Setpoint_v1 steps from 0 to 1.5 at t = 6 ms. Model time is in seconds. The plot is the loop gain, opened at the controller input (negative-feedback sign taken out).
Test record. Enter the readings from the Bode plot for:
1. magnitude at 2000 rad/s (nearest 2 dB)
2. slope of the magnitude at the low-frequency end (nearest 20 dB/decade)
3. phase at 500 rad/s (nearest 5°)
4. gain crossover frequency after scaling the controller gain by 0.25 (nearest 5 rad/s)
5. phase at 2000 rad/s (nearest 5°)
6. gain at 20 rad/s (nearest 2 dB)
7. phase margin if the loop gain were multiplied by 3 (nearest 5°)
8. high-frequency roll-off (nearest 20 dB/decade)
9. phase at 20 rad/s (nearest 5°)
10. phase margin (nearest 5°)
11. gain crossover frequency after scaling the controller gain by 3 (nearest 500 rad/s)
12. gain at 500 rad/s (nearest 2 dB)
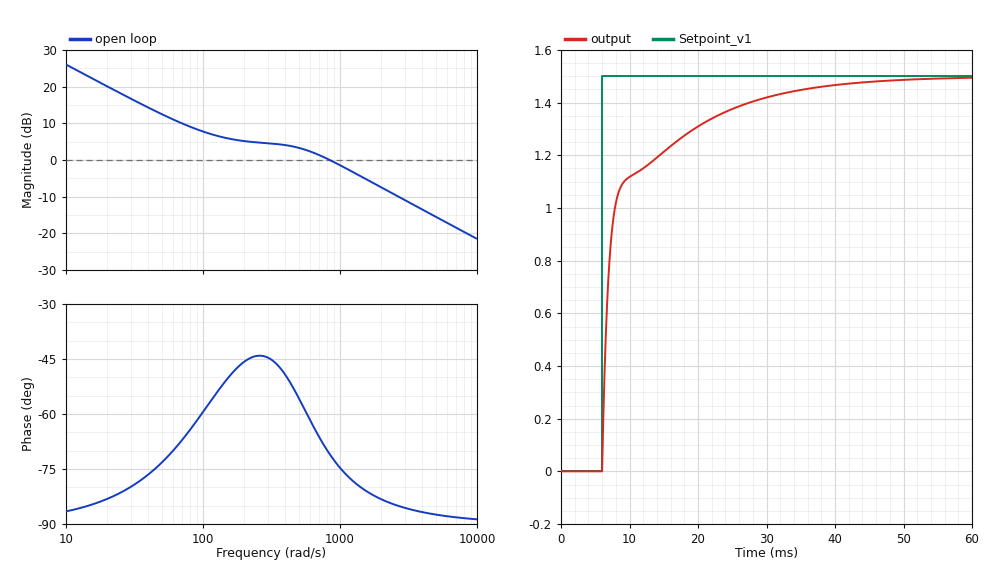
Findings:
-8 dB
-20 dB/decade
-55°
55 rad/s
-85°
20 dB
95°
-20 dB/decade
-85°
110°
2500 rad/s
4 dB
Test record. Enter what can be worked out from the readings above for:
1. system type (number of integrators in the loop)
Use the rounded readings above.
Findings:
1
